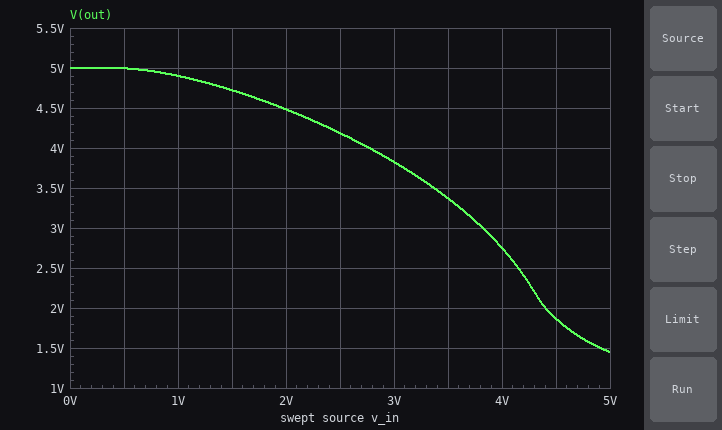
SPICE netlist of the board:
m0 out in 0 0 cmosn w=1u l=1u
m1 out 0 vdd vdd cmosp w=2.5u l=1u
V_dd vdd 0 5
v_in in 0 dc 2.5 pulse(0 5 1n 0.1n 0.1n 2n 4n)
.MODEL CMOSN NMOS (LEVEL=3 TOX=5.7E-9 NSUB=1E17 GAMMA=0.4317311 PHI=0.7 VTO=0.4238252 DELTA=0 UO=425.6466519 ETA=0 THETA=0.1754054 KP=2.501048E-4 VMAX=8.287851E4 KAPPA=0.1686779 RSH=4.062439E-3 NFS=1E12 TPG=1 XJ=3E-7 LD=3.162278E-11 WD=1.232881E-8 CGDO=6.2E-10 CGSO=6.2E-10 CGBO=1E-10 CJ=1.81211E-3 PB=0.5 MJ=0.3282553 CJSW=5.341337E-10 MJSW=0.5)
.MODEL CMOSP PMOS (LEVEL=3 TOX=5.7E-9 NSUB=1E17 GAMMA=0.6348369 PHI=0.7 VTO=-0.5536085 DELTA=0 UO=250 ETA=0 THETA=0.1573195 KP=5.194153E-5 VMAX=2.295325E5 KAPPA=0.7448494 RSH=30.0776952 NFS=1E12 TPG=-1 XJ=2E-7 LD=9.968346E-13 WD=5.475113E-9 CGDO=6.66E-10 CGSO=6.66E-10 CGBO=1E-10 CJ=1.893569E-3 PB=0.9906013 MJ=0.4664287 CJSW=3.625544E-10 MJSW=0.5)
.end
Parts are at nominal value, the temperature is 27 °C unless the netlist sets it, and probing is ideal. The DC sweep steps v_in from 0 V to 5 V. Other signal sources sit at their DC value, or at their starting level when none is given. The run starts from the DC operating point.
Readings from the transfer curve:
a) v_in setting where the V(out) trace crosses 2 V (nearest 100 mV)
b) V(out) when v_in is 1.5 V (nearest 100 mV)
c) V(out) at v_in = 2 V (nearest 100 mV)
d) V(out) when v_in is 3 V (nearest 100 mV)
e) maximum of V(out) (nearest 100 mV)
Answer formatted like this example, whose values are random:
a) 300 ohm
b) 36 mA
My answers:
a) 4.4 V
b) 4.7 V
c) 4.5 V
d) 3.8 V
e) 5.0 V
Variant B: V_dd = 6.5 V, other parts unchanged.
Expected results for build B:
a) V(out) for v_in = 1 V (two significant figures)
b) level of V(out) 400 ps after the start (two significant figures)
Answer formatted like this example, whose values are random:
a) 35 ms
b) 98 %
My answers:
a) 6.4 V
b) 6.5 V
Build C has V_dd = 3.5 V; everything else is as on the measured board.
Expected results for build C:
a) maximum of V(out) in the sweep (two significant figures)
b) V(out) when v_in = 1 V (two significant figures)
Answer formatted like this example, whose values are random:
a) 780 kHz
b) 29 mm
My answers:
a) 3.5 V
b) 3.4 V
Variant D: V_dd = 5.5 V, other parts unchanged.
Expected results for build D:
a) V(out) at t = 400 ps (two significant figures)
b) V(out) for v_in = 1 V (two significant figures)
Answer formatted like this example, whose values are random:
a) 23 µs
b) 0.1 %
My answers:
a) 5.5 V
b) 5.4 V
